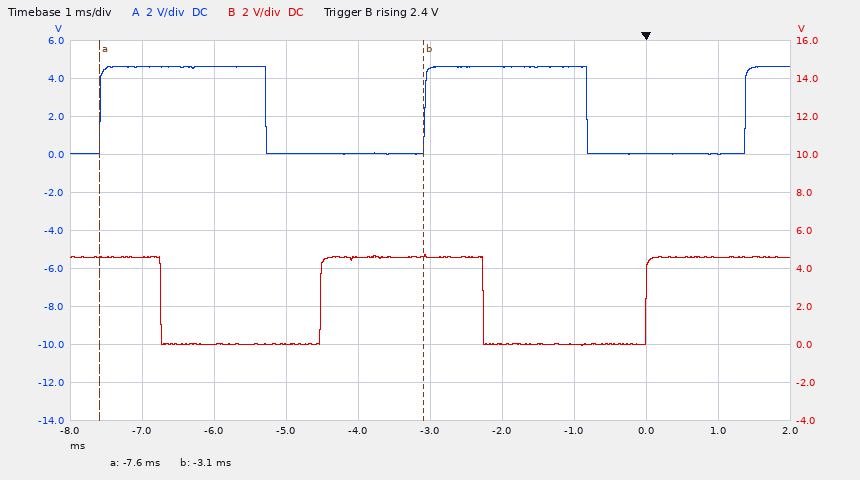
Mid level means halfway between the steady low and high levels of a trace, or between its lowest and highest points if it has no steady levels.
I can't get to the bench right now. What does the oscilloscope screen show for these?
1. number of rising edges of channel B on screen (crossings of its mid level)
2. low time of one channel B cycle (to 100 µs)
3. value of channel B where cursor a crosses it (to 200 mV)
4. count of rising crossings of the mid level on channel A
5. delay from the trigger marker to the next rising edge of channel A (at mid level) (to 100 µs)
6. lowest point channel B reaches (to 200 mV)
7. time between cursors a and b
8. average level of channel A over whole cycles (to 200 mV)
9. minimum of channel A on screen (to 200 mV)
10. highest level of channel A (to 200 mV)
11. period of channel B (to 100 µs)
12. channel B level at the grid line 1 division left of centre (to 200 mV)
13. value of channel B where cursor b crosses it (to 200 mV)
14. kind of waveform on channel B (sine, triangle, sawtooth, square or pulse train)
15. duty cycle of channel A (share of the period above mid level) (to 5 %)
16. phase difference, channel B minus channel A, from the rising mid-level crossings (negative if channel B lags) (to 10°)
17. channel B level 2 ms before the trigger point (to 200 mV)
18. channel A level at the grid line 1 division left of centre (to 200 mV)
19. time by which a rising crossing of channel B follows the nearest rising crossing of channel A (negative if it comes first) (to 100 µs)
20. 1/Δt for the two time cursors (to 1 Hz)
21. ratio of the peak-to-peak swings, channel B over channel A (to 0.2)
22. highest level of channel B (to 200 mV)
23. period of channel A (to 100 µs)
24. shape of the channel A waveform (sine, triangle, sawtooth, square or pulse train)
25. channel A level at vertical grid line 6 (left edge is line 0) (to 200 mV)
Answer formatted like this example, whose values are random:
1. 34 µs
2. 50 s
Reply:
1. 2
2. 2.3 ms
3. 4.6 V
4. 3
5. 1.4 ms
6. 0.0 V
7. 4.5 ms
8. 2.4 V
9. 0.0 V
10. 4.6 V
11. 4.5 ms
12. 4.6 V
13. 4.6 V
14. square
15. 50 %
16. +110°
17. 0.0 V
18. 0.0 V
19. -1.4 ms
20. 222 Hz
21. 1.0
22. 4.8 V
23. 4.5 ms
24. square
25. 4.6 V
